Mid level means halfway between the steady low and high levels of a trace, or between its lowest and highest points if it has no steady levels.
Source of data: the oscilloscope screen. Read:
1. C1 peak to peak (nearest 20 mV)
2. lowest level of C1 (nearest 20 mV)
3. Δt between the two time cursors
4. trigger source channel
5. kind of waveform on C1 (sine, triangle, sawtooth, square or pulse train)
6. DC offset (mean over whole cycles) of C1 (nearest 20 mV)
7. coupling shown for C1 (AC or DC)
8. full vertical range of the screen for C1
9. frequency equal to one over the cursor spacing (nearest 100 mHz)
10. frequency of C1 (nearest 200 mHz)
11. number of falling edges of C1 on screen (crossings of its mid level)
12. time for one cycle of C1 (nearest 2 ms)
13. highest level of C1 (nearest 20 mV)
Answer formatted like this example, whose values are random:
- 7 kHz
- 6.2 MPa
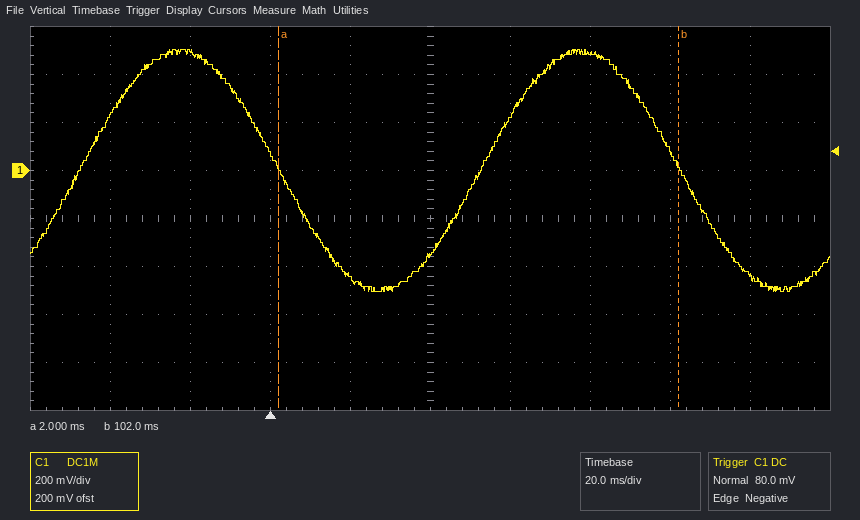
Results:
- 1.00 V
- -500 mV
- 100 ms
- C1
- sine
- 0 mV
- DC
- 1.6 V
- 10.0 Hz
- 10.0 Hz
- 2
- 100 ms
- 500 mV
